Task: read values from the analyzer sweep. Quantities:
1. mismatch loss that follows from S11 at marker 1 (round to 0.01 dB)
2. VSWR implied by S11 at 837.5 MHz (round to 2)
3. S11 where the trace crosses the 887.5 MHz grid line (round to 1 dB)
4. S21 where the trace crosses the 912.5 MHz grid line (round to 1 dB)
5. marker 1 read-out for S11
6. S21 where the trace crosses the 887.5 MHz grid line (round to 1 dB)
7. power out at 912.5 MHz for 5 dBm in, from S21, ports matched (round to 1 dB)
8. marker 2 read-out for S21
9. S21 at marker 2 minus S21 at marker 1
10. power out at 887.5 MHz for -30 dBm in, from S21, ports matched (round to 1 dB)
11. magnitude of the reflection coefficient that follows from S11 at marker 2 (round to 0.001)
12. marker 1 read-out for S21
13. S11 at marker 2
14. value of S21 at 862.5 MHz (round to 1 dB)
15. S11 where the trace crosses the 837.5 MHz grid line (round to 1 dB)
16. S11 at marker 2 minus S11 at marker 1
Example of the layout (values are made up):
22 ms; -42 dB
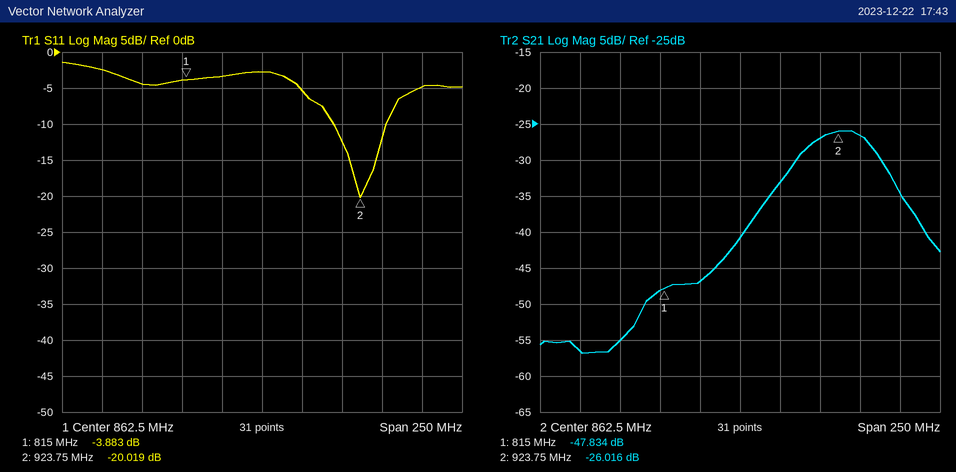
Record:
2.28 dB; 6; -5 dB; -27 dB; -3.883 dB; -33 dB; -22 dBm; -26.016 dB; 21.818 dB; -63 dBm; 0.100; -47.834 dB; -20.019 dB; -41 dB; -3 dB; -16.136 dB
